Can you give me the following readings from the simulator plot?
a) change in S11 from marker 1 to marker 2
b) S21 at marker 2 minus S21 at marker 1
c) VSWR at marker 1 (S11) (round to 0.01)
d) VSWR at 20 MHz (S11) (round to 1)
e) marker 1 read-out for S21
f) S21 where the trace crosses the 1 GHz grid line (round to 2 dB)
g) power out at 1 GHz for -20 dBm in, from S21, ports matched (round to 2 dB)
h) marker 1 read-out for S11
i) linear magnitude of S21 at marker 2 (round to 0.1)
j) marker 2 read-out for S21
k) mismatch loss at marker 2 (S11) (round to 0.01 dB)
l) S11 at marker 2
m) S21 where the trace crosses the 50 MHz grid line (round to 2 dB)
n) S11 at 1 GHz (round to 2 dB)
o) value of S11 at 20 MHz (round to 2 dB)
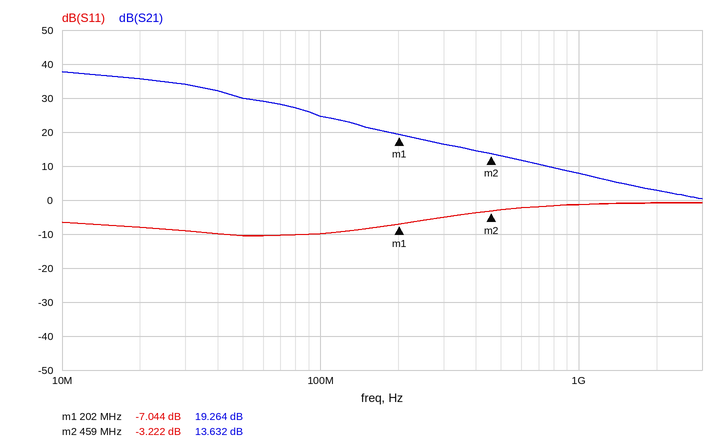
3.822 dB
-5.632 dB
2.60
2
19.264 dB
8 dB
-12 dBm
-7.044 dB
4.8
13.632 dB
2.81 dB
-3.222 dB
30 dB
-2 dB
-8 dB
